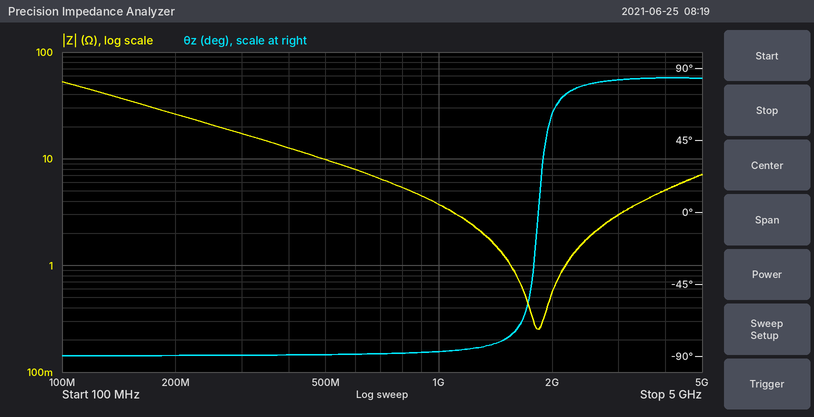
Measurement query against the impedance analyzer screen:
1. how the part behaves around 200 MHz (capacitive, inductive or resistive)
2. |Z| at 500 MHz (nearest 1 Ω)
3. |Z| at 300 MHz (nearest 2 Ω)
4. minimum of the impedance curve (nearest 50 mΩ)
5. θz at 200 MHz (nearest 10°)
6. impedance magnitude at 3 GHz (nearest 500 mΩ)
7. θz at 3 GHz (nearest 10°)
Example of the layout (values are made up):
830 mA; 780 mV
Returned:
capacitive; 10 Ω; 18 Ω; 250 mΩ; -90°; 3.0 Ω; 80°
